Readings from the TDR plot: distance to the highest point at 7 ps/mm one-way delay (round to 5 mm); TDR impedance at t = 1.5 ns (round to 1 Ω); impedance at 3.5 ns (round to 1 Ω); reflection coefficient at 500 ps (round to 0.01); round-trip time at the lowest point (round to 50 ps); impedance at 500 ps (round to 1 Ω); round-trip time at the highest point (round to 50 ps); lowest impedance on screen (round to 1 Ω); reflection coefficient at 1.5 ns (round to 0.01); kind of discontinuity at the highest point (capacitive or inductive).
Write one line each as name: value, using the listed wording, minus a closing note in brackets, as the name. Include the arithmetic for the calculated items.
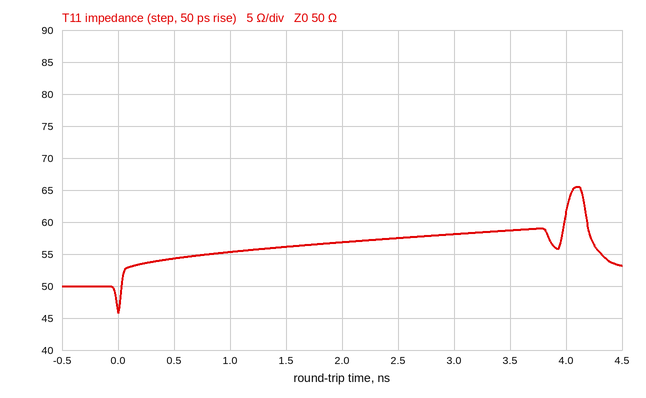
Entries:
distance to the highest point at 7 ps/mm one-way delay: 4.10 ns / 2 / 7 ps/mm ≈ 293 mm, so 295 mm to the nearest 5 mm
TDR impedance at t = 1.5 ns: 56 Ω
impedance at 3.5 ns: 59 Ω
reflection coefficient at 500 ps: (54 − 50)/(54 + 50) ≈ +0.04
round-trip time at the lowest point: 0 ps
impedance at 500 ps: 54 Ω
round-trip time at the highest point: 4.10 ns
lowest impedance on screen: 46 Ω
reflection coefficient at 1.5 ns: (56 − 50)/(56 + 50) ≈ +0.06
kind of discontinuity at the highest point: inductive
